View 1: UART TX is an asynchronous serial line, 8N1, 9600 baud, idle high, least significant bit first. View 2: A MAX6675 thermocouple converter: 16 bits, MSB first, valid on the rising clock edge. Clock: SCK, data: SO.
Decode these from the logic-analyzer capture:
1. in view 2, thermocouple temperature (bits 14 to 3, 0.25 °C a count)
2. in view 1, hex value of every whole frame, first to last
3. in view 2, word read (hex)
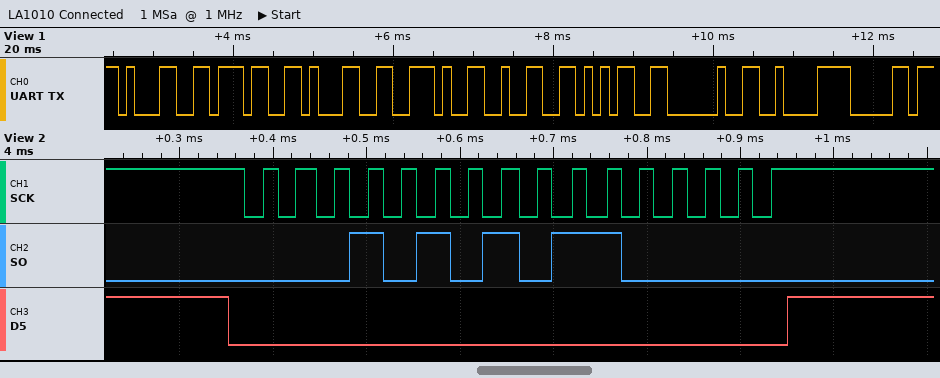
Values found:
171.00 °C
31 37 31 2E 32 35 20 C2 B0
0x1560
